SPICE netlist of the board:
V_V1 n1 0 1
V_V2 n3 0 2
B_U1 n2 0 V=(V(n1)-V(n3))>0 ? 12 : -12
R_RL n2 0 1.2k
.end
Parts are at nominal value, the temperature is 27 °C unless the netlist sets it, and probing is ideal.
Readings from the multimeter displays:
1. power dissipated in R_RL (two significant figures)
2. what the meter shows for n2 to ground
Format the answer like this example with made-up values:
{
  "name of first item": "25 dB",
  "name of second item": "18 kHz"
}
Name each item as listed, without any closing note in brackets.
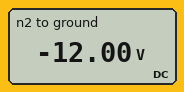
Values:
{
  "power dissipated in R_RL": "120 mW",
  "what the meter shows for n2 to ground": "-12.00 V"
}
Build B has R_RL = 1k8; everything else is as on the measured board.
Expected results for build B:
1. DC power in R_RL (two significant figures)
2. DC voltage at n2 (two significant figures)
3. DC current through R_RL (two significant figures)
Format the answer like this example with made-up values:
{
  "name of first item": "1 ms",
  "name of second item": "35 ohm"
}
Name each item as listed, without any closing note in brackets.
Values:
{
  "DC power in R_RL": "80 mW",
  "DC voltage at n2": "-12 V",
  "DC current through R_RL": "6.7 mA"
}
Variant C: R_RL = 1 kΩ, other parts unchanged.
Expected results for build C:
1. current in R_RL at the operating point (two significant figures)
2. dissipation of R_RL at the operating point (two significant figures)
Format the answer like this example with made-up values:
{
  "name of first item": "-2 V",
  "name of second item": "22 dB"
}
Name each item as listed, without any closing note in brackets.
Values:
{
  "current in R_RL at the operating point": "12 mA",
  "dissipation of R_RL at the operating point": "140 mW"
}
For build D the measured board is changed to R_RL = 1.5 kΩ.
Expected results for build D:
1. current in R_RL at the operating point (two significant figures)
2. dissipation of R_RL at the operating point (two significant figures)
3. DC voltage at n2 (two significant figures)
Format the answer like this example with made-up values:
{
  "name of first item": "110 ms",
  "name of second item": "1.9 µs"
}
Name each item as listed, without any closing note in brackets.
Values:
{
  "current in R_RL at the operating point": "8.0 mA",
  "dissipation of R_RL at the operating point": "96 mW",
  "DC voltage at n2": "-12 V"
}
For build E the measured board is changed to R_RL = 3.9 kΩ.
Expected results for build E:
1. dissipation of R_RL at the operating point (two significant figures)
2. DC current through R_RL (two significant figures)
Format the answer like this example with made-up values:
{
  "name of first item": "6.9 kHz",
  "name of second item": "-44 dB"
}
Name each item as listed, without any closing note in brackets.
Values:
{
  "dissipation of R_RL at the operating point": "37 mW",
  "DC current through R_RL": "3.1 mA"
}
